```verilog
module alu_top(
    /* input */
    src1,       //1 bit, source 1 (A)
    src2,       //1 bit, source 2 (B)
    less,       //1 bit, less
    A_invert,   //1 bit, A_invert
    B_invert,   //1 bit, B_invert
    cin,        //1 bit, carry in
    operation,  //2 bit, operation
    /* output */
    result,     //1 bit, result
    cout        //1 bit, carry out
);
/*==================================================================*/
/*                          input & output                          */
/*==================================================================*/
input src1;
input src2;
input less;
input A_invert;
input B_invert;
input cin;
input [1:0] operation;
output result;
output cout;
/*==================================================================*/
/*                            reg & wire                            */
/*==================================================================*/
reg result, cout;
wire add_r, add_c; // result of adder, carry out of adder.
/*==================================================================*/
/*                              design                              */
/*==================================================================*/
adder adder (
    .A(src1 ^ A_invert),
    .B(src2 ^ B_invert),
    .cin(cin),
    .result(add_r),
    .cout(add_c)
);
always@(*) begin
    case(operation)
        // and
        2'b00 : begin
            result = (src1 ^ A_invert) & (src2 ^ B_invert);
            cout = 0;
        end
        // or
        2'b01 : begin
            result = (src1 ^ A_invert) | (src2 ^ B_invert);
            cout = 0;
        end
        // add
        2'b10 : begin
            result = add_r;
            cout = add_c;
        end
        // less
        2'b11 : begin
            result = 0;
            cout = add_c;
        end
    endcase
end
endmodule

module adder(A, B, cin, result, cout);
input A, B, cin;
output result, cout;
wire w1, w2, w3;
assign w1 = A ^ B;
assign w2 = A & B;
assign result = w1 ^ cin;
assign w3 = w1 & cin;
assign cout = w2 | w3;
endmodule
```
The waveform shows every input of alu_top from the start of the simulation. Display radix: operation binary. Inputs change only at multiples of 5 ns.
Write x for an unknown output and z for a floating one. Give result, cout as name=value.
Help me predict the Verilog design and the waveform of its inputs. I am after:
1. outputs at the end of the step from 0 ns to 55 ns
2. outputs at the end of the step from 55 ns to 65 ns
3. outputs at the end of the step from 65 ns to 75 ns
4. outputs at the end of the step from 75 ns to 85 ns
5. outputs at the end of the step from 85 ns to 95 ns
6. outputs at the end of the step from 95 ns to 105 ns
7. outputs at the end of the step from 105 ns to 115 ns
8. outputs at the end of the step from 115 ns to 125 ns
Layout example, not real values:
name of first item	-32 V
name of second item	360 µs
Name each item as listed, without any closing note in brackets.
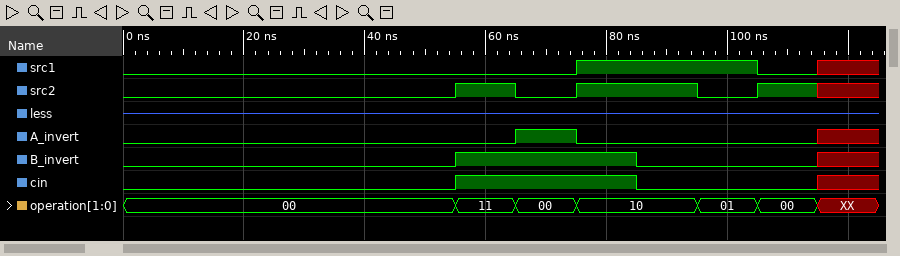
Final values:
outputs at the end of the step from 0 ns to 55 ns	result=0, cout=0
outputs at the end of the step from 55 ns to 65 ns	result=0, cout=0
outputs at the end of the step from 65 ns to 75 ns	result=1, cout=0
outputs at the end of the step from 75 ns to 85 ns	result=0, cout=1
outputs at the end of the step from 85 ns to 95 ns	result=0, cout=1
outputs at the end of the step from 95 ns to 105 ns	result=1, cout=0
outputs at the end of the step from 105 ns to 115 ns	result=0, cout=0
outputs at the end of the step from 115 ns to 125 ns	result=0, cout=0
